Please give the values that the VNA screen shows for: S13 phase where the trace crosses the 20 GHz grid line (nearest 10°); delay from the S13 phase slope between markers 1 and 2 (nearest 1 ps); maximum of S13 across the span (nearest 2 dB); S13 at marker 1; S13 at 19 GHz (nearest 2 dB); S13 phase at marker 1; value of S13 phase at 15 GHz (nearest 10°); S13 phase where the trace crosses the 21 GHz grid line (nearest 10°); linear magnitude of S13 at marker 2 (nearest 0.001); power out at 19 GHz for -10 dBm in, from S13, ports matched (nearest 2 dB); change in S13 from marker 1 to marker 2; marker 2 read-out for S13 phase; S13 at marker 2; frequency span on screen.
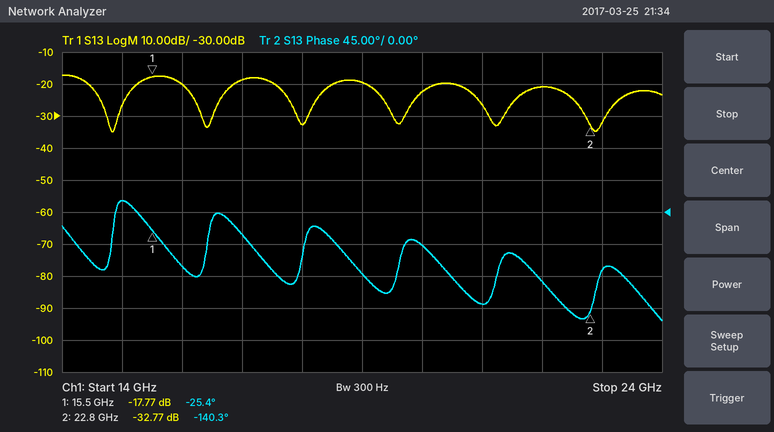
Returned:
-50°
44 ps
-18 dB
-17.77 dB
-20 dB
-25.4°
20°
-130°
0.023
-30 dBm
-15.00 dB
-140.3°
-32.77 dB
10 GHz
